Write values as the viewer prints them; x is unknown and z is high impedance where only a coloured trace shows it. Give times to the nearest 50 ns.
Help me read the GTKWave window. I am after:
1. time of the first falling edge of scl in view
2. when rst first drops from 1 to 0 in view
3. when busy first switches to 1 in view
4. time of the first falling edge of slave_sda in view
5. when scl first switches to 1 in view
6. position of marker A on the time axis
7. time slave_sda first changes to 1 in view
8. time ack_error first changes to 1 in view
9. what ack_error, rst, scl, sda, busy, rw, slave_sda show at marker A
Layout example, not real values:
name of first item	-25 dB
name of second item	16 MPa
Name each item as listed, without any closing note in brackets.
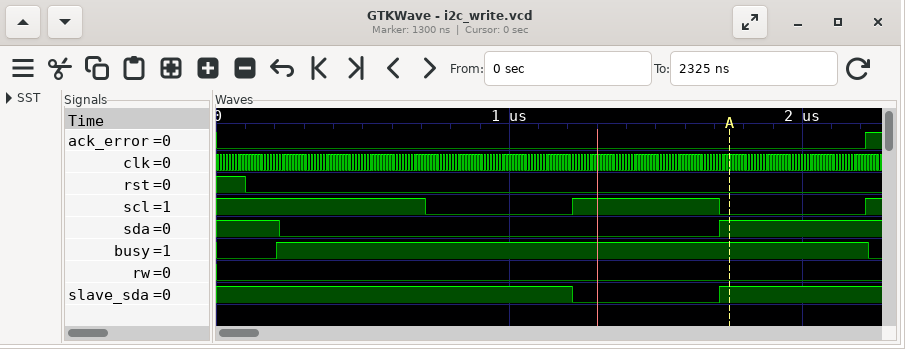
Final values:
time of the first falling edge of scl in view	700 ns
when rst first drops from 1 to 0 in view	100 ns
when busy first switches to 1 in view	200 ns
time of the first falling edge of slave_sda in view	1200 ns
when scl first switches to 1 in view	1200 ns
position of marker A on the time axis	1750 ns
time slave_sda first changes to 1 in view	1700 ns
time ack_error first changes to 1 in view	2200 ns
what ack_error, rst, scl, sda, busy, rw, slave_sda show at marker A	ack_error=0, rst=0, scl=0, sda=1, busy=1, rw=0, slave_sda=1
